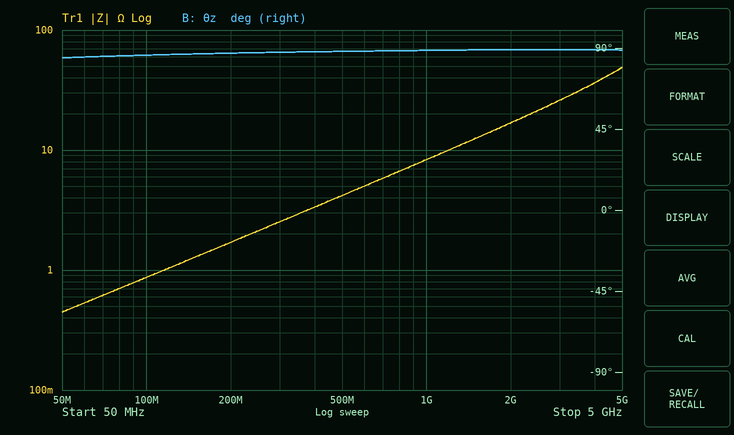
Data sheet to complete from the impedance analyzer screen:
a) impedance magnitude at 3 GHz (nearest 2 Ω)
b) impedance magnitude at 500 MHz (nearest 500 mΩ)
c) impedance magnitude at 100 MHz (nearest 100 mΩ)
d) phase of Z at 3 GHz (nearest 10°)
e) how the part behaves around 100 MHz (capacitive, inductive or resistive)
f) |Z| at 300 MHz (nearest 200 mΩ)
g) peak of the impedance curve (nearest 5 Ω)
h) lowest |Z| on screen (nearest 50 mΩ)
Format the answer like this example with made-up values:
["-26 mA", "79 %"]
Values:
["26 Ω", "4.0 Ω", "900 mΩ", "90°", "inductive", "2.6 Ω", "50 Ω", "450 mΩ"]
